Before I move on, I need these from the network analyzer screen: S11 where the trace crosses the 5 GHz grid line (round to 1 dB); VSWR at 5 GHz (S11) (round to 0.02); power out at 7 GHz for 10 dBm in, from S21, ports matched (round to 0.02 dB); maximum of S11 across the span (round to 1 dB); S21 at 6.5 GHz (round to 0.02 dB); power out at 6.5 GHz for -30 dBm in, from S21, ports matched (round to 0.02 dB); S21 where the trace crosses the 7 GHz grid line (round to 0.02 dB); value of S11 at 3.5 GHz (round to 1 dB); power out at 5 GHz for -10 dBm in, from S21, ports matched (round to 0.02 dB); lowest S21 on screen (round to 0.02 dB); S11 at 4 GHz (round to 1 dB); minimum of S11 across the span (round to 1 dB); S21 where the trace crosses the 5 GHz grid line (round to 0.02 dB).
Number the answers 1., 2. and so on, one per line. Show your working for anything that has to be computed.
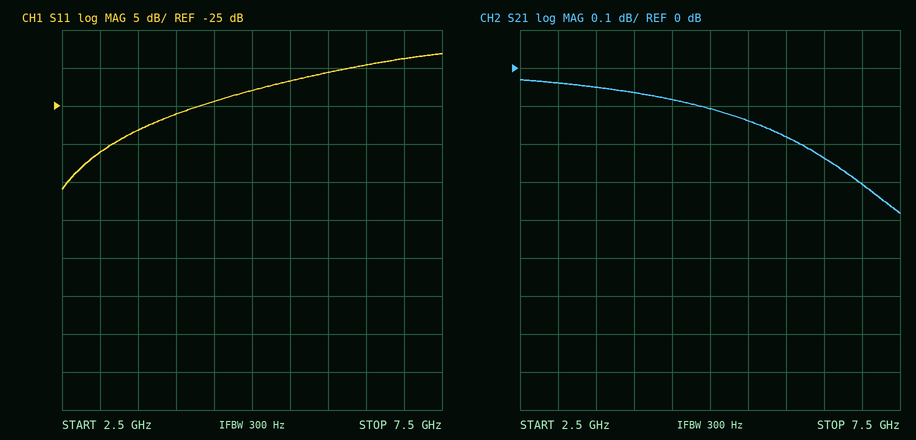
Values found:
1. -23 dB
2. |Γ| = 10^(-23/20) = 0.0708; VSWR = (1 + 0.0708)/(1 − 0.0708) ≈ 1.15, so 1.16 to the nearest 0.02
3. 10 dBm + (-0.30 dB) = 9.70 dBm
4. -18 dB
5. -0.24 dB
6. -30 dBm + (-0.24 dB) = -30.24 dBm
7. -0.30 dB
8. -28 dB
9. -10 dBm + (-0.10 dB) = -10.10 dBm
10. -0.38 dB
11. -26 dB
12. -36 dB
13. -0.10 dB
